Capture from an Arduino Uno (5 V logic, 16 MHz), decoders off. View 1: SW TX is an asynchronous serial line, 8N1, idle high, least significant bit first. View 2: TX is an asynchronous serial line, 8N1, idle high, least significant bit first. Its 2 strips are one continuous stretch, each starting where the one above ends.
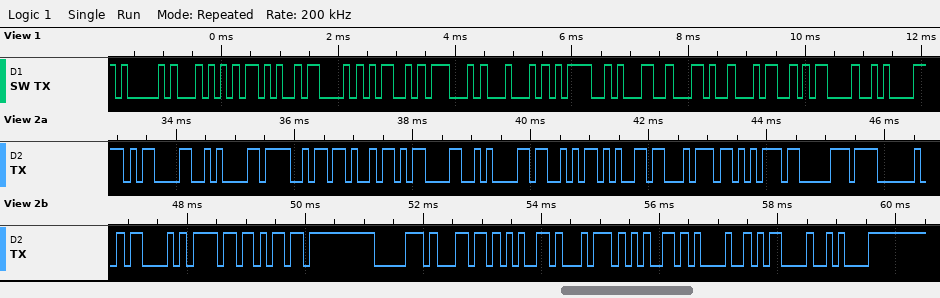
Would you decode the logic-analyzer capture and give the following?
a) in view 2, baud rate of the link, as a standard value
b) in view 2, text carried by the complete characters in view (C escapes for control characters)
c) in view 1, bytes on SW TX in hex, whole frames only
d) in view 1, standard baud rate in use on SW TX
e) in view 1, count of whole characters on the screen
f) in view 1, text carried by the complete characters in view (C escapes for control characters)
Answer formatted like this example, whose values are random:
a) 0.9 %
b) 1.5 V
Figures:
a) 9600 baud
b) "\r\nOK\r\nSetup Complete!\r\n"
c) 41 54 2B 43 4D 47 44 3D 31 2C 34 0D 0A
d) 9600 baud
e) 13
f) "AT+CMGD=1,4\r\n"
